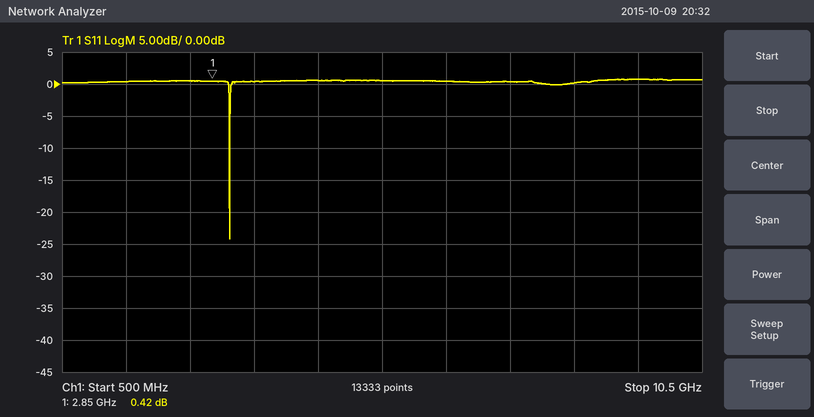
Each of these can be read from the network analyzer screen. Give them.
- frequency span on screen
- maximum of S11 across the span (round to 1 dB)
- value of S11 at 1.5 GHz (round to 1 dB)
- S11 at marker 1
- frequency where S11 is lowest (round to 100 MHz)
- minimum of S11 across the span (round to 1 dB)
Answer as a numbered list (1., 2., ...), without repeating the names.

1. 10 GHz
2. 1 dB
3. 0 dB
4. 0.42 dB
5. 3.1 GHz
6. -24 dB
